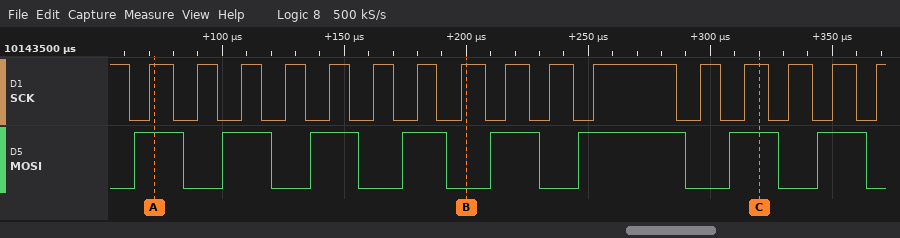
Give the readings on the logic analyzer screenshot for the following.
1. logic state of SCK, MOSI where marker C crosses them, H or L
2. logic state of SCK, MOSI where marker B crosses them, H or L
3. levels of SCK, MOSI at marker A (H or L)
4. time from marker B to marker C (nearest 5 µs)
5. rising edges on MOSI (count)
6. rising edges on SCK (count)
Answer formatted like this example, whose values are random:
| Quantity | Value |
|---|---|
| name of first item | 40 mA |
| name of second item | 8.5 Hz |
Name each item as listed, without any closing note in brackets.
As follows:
| Quantity | Value |
|---|---|
| logic state of SCK, MOSI where marker C crosses them, H or L | SCK=H, MOSI=H |
| logic state of SCK, MOSI where marker B crosses them, H or L | SCK=H, MOSI=L |
| levels of SCK, MOSI at marker A | SCK=H, MOSI=H |
| time from marker B to marker C | 120 µs |
| rising edges on MOSI | 8 |
| rising edges on SCK | 16 |
